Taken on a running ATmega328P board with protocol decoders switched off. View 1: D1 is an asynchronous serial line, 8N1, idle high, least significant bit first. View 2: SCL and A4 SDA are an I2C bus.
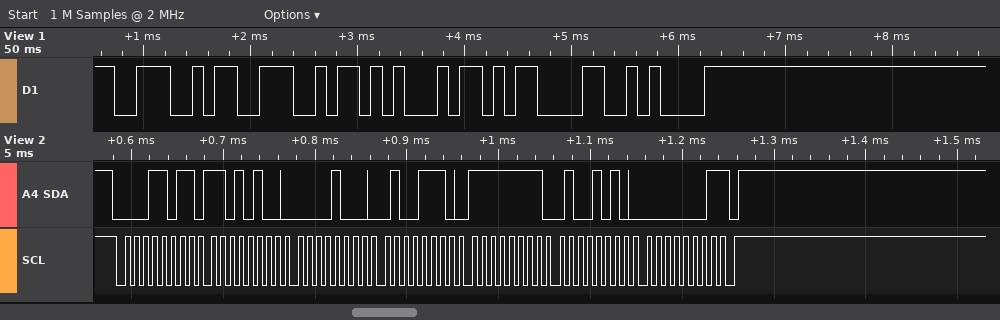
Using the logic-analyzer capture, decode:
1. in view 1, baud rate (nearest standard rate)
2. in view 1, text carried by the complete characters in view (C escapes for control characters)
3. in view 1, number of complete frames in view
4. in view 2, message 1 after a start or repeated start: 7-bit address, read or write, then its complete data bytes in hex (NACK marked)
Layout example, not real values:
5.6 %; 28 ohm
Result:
9600 baud; "NNE\r\n"; 5; 0x0D read: D4 08 4E FF 4A 01 NACK
